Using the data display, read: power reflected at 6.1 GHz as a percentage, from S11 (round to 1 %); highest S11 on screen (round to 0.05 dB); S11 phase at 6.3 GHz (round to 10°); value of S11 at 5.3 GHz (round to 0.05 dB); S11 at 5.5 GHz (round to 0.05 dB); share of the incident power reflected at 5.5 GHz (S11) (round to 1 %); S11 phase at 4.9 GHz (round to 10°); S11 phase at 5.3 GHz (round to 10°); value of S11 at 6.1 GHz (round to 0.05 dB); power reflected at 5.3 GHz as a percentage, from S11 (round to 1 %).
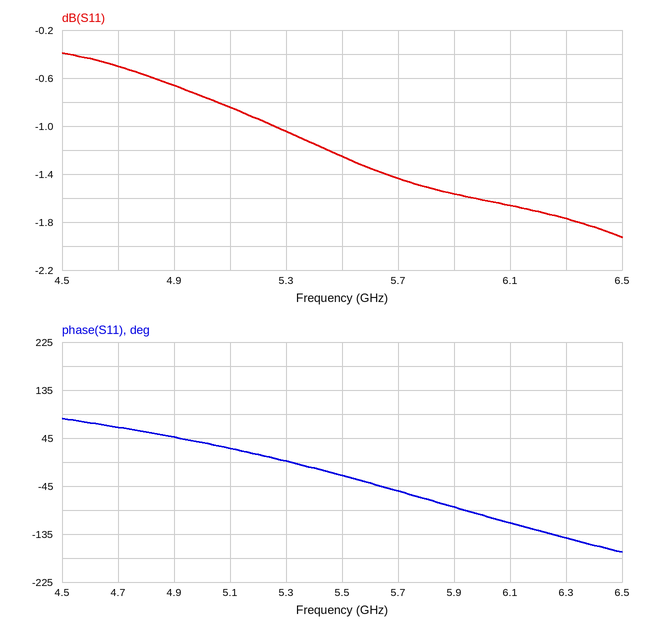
68 %
-0.40 dB
-140°
-1.05 dB
-1.25 dB
75 %
50°
0°
-1.65 dB
79 %
